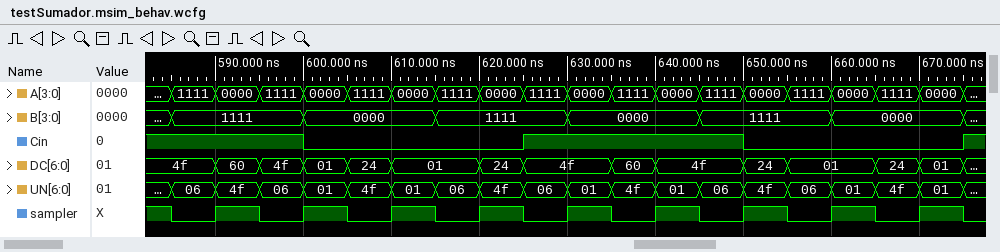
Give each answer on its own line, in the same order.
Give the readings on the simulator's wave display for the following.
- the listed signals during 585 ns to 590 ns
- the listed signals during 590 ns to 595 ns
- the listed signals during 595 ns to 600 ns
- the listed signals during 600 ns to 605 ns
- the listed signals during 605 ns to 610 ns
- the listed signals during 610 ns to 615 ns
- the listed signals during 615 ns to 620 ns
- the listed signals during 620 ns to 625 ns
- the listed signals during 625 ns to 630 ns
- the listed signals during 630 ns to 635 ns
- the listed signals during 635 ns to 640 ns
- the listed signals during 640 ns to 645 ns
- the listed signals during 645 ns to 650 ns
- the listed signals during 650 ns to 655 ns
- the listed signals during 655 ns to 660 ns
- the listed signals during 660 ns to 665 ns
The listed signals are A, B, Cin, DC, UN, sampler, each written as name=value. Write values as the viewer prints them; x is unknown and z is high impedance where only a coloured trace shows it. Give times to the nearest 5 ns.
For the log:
A=1111, B=1111, Cin=1, DC=4f, UN=06, sampler=0
A=0000, B=1111, Cin=1, DC=60, UN=4f, sampler=1
A=1111, B=1111, Cin=1, DC=4f, UN=06, sampler=0
A=0000, B=0000, Cin=0, DC=01, UN=01, sampler=1
A=1111, B=0000, Cin=0, DC=24, UN=4f, sampler=0
A=0000, B=0000, Cin=0, DC=01, UN=01, sampler=1
A=1111, B=1111, Cin=0, DC=01, UN=06, sampler=0
A=0000, B=1111, Cin=0, DC=24, UN=4f, sampler=1
A=1111, B=1111, Cin=1, DC=4f, UN=06, sampler=0
A=0000, B=0000, Cin=1, DC=4f, UN=01, sampler=1
A=1111, B=0000, Cin=1, DC=60, UN=4f, sampler=0
A=0000, B=0000, Cin=1, DC=4f, UN=01, sampler=1
A=1111, B=1111, Cin=1, DC=4f, UN=06, sampler=0
A=0000, B=1111, Cin=0, DC=24, UN=4f, sampler=1
A=1111, B=1111, Cin=0, DC=01, UN=06, sampler=0
A=0000, B=0000, Cin=0, DC=01, UN=01, sampler=1
